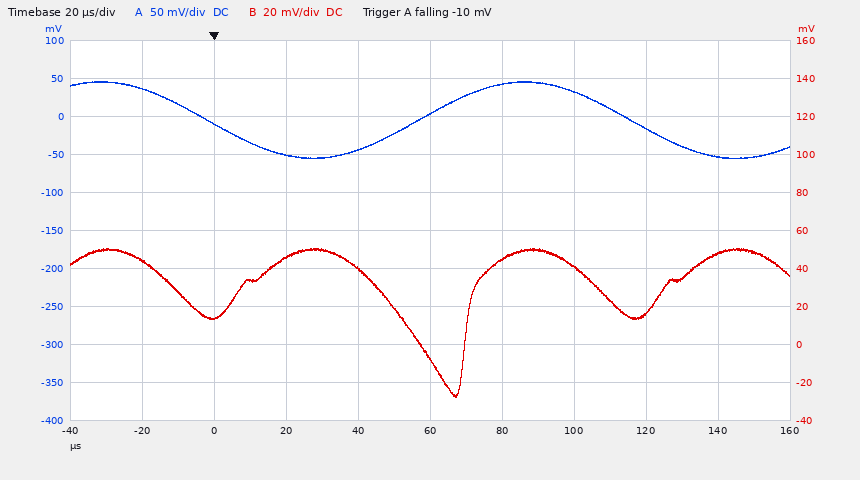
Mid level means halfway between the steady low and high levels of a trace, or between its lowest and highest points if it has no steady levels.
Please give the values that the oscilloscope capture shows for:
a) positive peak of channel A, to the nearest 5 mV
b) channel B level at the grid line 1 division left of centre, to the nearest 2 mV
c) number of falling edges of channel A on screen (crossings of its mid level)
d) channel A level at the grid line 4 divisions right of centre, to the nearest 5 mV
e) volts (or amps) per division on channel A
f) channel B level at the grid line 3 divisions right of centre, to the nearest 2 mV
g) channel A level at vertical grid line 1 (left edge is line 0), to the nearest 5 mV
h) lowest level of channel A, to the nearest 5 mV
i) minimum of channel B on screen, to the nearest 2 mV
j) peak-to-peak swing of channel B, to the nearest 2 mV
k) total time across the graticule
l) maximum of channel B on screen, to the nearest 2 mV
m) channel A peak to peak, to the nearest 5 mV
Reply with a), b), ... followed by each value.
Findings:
a) 45 mV
b) 40 mV
c) 2
d) -55 mV
e) 50 mV
f) 16 mV
g) 35 mV
h) -55 mV
i) -28 mV
j) 78 mV
k) 200 µs
l) 50 mV
m) 100 mV
